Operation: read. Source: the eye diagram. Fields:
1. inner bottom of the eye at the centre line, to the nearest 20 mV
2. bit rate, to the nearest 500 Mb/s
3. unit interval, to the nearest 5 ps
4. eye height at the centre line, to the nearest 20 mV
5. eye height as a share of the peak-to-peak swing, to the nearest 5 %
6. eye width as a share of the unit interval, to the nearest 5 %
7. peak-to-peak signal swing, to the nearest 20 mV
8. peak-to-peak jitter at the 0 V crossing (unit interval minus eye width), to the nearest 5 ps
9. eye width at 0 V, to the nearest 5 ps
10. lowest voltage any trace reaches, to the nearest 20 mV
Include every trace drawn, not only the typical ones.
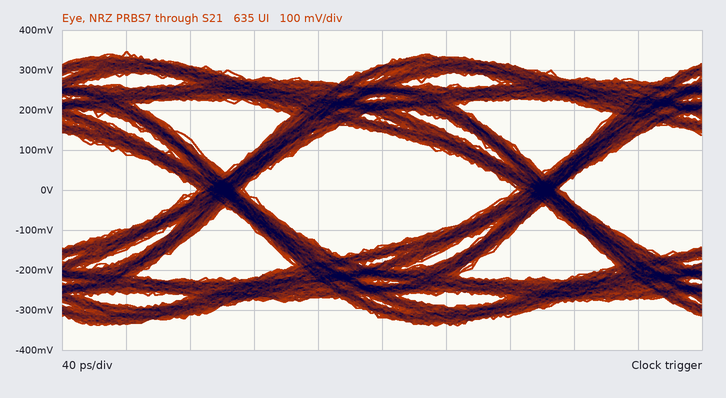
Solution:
-140 mV
5.0 Gb/s
200 ps
280 mV
40 %
85 %
680 mV
30 ps
170 ps
-340 mV
